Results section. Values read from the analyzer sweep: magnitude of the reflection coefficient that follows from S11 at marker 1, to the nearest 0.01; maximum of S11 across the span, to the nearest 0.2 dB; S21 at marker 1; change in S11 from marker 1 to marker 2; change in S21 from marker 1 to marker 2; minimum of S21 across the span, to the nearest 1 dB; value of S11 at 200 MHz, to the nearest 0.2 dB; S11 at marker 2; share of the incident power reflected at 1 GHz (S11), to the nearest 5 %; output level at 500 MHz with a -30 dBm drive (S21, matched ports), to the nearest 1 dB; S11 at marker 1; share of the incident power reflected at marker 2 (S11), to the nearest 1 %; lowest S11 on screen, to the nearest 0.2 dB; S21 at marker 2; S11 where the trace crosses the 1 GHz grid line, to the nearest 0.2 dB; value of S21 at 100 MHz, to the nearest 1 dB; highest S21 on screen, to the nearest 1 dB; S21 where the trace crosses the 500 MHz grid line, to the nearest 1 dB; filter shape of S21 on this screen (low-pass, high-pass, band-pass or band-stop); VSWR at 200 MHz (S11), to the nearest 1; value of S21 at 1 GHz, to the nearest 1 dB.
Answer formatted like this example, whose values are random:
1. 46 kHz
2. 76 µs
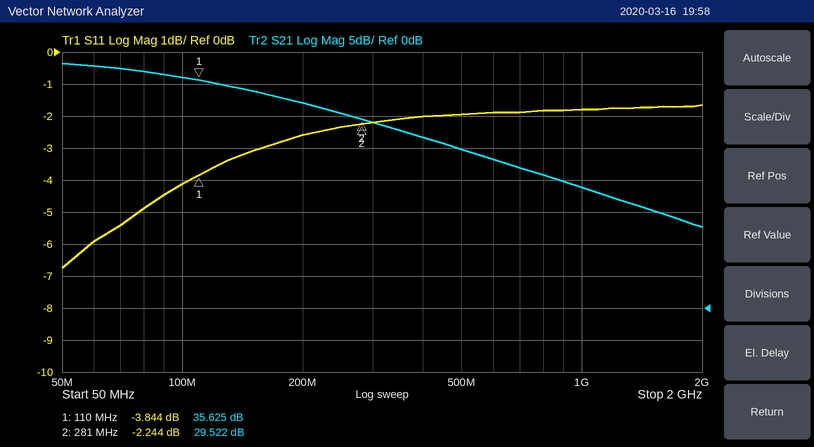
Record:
1. 0.64
2. -1.6 dB
3. 35.625 dB
4. 1.600 dB
5. -6.103 dB
6. 13 dB
7. -2.6 dB
8. -2.244 dB
9. 65 %
10. -5 dBm
11. -3.844 dB
12. 60 %
13. -6.8 dB
14. 29.522 dB
15. -1.8 dB
16. 36 dB
17. 38 dB
18. 25 dB
19. low-pass
20. 7
21. 19 dB
